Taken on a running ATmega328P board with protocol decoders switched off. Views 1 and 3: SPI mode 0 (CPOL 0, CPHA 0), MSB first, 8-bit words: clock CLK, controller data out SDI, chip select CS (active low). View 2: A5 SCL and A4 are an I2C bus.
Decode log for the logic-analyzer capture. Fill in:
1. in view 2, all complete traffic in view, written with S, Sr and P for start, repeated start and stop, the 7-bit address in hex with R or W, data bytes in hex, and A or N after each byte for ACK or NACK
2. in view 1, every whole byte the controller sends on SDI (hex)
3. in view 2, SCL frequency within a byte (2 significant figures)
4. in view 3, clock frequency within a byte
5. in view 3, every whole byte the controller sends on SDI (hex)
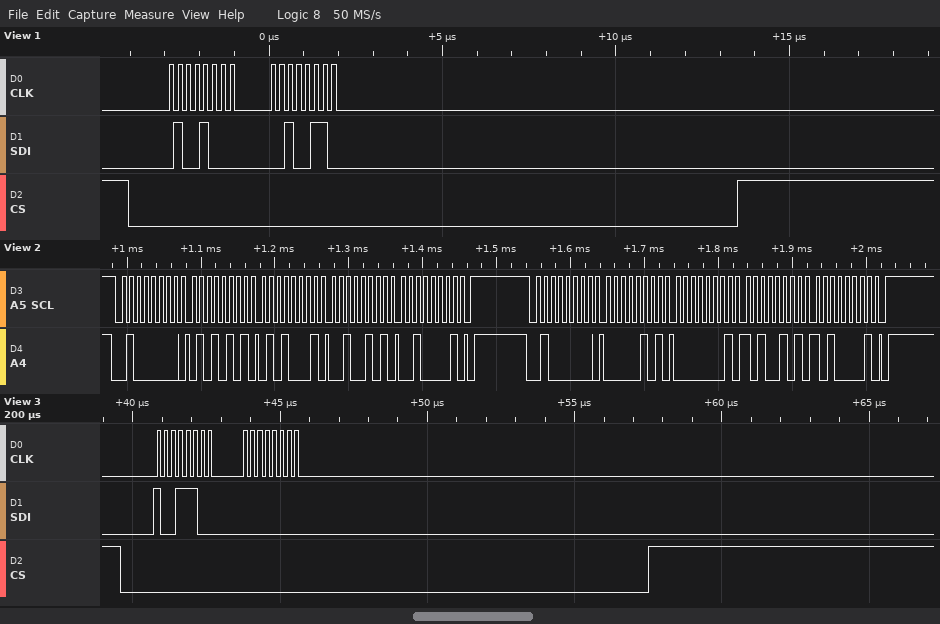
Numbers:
S 20W A 55 A 51 A 25 A 21 A P S 20W A 05 A 01 A A5 A A1 A P
48 26
100 kHz
4 MHz
9C 00
